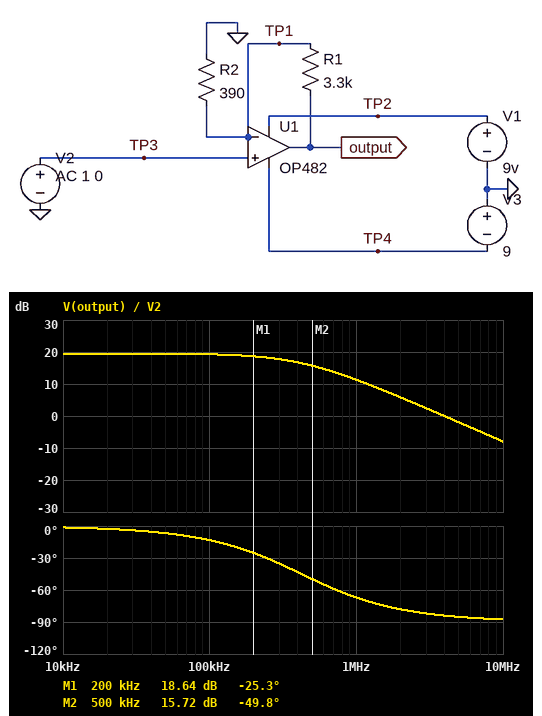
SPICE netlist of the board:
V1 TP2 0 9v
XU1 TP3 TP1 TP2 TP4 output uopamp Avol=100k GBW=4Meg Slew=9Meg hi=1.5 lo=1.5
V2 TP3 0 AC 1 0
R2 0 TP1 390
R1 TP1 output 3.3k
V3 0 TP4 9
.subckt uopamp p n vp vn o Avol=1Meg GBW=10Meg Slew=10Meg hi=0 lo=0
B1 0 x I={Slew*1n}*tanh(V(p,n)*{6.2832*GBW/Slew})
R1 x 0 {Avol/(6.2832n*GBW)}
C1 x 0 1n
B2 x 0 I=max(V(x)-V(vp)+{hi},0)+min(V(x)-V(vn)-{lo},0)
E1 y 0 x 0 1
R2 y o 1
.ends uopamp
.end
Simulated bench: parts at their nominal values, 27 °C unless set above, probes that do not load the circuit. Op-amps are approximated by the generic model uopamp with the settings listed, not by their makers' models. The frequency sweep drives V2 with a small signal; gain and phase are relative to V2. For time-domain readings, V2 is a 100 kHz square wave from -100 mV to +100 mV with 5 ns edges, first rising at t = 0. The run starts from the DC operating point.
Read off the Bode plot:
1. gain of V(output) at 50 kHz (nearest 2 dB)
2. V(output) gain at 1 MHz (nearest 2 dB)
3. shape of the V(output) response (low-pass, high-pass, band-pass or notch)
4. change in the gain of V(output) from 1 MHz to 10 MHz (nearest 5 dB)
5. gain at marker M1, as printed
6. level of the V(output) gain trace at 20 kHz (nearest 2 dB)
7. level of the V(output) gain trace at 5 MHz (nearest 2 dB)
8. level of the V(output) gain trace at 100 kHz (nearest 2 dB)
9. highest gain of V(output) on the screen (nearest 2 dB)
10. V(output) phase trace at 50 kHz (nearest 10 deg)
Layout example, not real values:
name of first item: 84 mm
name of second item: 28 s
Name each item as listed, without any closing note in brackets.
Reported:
gain of V(output) at 50 kHz: 20 dB
V(output) gain at 1 MHz: 12 dB
shape of the V(output) response: low-pass
change in the gain of V(output) from 1 MHz to 10 MHz: -20 dB
gain at marker M1, as printed: 18.64 dB
level of the V(output) gain trace at 20 kHz: 20 dB
level of the V(output) gain trace at 5 MHz: -2 dB
level of the V(output) gain trace at 100 kHz: 20 dB
highest gain of V(output) on the screen: 20 dB
V(output) phase trace at 50 kHz: -10 deg
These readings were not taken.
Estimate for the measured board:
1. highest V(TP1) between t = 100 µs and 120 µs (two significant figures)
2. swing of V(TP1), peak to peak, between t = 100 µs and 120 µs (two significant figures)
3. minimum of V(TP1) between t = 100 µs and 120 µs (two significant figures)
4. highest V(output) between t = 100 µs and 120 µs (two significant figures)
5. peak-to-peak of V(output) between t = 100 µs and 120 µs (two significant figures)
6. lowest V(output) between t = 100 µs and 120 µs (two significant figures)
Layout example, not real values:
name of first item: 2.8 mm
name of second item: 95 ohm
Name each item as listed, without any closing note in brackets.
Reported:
highest V(TP1) between t = 100 µs and 120 µs: 100 mV
swing of V(TP1), peak to peak, between t = 100 µs and 120 µs: 200 mV
minimum of V(TP1) between t = 100 µs and 120 µs: -100 mV
highest V(output) between t = 100 µs and 120 µs: 950 mV
peak-to-peak of V(output) between t = 100 µs and 120 µs: 1.9 V
lowest V(output) between t = 100 µs and 120 µs: -950 mV
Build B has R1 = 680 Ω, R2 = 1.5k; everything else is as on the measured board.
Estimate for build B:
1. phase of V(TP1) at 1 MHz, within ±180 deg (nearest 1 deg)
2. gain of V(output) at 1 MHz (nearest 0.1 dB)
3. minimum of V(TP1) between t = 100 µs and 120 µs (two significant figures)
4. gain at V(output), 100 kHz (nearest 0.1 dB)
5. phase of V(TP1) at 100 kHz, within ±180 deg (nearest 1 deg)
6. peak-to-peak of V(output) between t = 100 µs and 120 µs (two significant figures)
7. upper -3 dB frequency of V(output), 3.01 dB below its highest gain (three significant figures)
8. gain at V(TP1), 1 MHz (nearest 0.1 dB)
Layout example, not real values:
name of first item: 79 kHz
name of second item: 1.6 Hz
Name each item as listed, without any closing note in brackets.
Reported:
phase of V(TP1) at 1 MHz, within ±180 deg: -20 deg
gain of V(output) at 1 MHz: 2.7 dB
minimum of V(TP1) between t = 100 µs and 120 µs: -100 mV
gain at V(output), 100 kHz: 3.2 dB
phase of V(TP1) at 100 kHz, within ±180 deg: -2 deg
peak-to-peak of V(output) between t = 100 µs and 120 µs: 290 mV
upper -3 dB frequency of V(output), 3.01 dB below its highest gain: 2.75 MHz
gain at V(TP1), 1 MHz: -0.5 dB
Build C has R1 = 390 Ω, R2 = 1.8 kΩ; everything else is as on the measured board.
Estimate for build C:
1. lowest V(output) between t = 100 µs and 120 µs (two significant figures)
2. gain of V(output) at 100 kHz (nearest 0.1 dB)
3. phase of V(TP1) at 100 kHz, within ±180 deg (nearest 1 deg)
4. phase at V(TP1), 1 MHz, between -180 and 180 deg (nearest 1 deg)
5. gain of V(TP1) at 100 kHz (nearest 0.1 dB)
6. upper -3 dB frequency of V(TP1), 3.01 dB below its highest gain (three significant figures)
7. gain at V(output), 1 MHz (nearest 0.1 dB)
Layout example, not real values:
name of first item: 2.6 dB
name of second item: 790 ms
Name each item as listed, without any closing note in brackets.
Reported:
lowest V(output) between t = 100 µs and 120 µs: -120 mV
gain of V(output) at 100 kHz: 1.7 dB
phase of V(TP1) at 100 kHz, within ±180 deg: -2 deg
phase at V(TP1), 1 MHz, between -180 and 180 deg: -17 deg
gain of V(TP1) at 100 kHz: 0 dB
upper -3 dB frequency of V(TP1), 3.01 dB below its highest gain: 3.29 MHz
gain at V(output), 1 MHz: 1.3 dB
